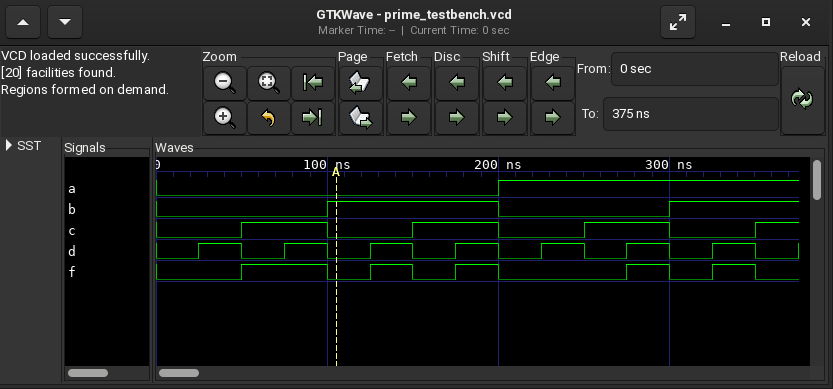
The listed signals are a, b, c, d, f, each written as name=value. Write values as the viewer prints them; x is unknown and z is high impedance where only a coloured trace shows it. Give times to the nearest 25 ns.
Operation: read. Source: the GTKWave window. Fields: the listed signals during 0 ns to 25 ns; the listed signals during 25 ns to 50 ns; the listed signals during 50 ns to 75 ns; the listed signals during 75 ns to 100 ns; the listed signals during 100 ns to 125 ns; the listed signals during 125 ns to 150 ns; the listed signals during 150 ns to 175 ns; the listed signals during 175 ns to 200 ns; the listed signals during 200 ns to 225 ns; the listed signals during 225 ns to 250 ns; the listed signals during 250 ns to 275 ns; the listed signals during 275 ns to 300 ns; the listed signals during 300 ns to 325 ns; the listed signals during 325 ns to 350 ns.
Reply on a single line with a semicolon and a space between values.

a=0, b=0, c=0, d=0, f=0; a=0, b=0, c=0, d=1, f=0; a=0, b=0, c=1, d=0, f=1; a=0, b=0, c=1, d=1, f=1; a=0, b=1, c=0, d=0, f=0; a=0, b=1, c=0, d=1, f=1; a=0, b=1, c=1, d=0, f=0; a=0, b=1, c=1, d=1, f=1; a=1, b=0, c=0, d=0, f=0; a=1, b=0, c=0, d=1, f=0; a=1, b=0, c=1, d=0, f=0; a=1, b=0, c=1, d=1, f=1; a=1, b=1, c=0, d=0, f=0; a=1, b=1, c=0, d=1, f=1
